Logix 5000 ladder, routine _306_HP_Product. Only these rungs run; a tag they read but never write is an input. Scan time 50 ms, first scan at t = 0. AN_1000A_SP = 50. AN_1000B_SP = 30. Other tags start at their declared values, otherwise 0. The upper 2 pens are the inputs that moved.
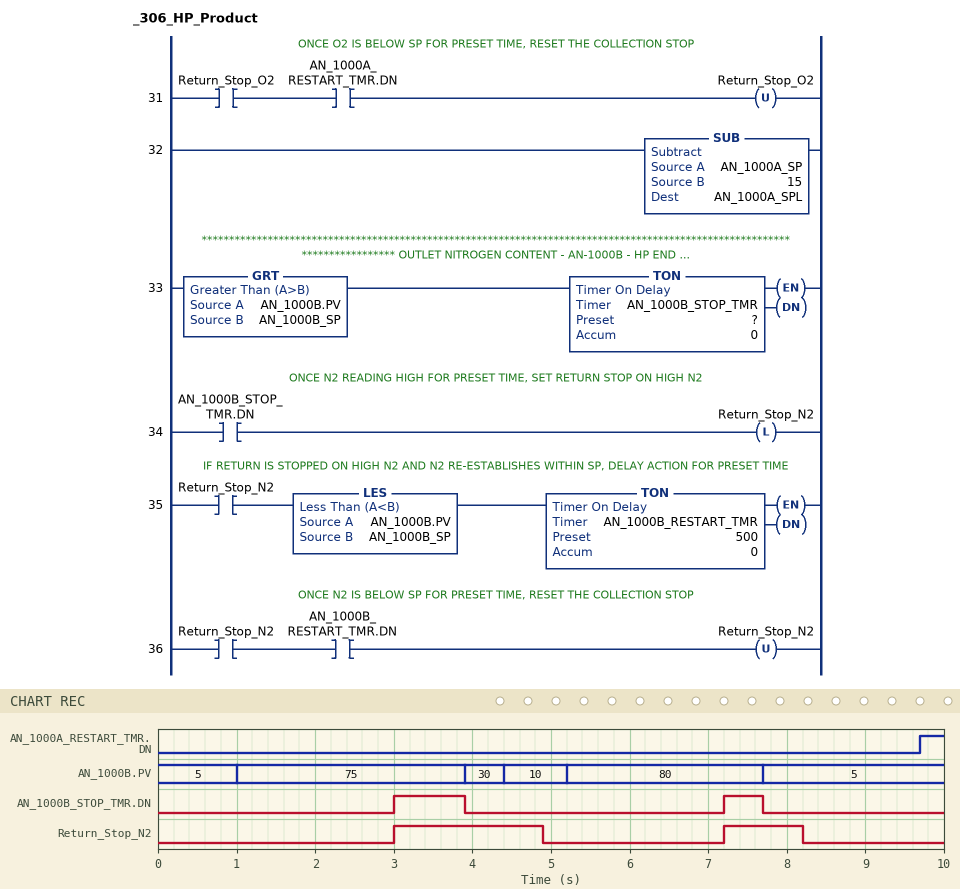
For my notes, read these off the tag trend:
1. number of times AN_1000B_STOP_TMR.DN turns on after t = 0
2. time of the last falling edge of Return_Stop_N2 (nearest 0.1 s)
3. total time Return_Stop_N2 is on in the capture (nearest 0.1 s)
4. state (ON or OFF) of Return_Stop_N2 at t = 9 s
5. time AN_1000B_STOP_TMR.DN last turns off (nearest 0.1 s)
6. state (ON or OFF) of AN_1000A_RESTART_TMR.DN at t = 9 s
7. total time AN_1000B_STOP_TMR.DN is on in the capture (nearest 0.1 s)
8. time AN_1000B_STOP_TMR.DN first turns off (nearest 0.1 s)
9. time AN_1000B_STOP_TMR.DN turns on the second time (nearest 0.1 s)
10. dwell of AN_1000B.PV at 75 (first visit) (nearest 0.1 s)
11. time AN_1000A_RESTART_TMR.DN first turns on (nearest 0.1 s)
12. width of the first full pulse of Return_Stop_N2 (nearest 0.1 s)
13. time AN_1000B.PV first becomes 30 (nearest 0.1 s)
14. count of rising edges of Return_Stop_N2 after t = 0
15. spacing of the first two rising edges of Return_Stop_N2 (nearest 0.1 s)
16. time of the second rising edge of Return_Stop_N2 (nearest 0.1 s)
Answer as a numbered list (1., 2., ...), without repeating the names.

1. 2
2. 8.2 s
3. 2.9 s
4. OFF
5. 7.7 s
6. OFF
7. 1.4 s
8. 3.9 s
9. 7.2 s
10. 2.9 s
11. 9.7 s
12. 1.9 s
13. 3.9 s
14. 2
15. 4.2 s
16. 7.2 s
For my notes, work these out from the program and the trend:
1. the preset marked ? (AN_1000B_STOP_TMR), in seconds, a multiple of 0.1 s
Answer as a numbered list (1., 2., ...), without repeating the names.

1. 2.0 s
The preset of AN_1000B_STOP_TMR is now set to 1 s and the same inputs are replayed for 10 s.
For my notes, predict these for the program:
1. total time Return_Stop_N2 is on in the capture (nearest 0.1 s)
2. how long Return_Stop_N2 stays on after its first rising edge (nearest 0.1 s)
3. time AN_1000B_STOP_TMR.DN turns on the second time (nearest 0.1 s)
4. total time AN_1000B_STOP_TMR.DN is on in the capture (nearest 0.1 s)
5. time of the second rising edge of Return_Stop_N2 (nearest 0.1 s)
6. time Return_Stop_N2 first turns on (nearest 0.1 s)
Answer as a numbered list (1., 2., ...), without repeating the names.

1. 4.9 s
2. 2.9 s
3. 6.2 s
4. 3.4 s
5. 6.2 s
6. 2.0 s
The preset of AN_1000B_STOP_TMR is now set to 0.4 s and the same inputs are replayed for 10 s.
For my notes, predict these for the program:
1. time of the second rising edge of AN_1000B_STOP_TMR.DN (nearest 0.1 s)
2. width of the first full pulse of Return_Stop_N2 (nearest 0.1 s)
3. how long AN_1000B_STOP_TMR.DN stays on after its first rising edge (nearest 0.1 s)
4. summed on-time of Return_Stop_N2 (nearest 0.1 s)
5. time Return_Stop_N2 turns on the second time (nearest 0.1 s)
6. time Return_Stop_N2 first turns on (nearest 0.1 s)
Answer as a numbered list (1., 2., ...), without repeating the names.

1. 5.6 s
2. 3.5 s
3. 2.5 s
4. 6.1 s
5. 5.6 s
6. 1.4 s
